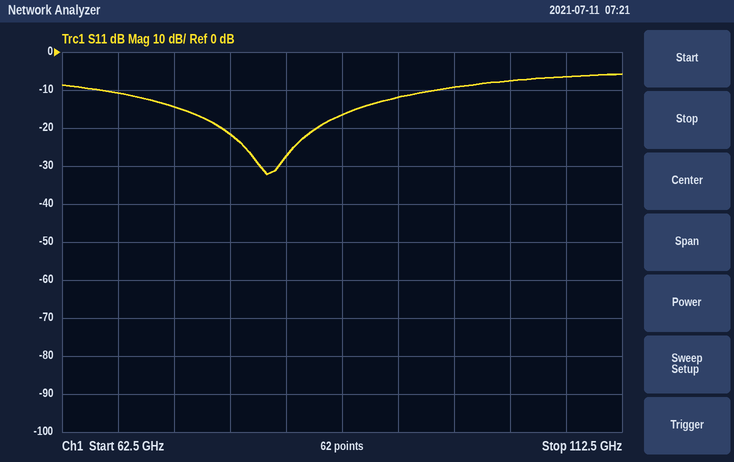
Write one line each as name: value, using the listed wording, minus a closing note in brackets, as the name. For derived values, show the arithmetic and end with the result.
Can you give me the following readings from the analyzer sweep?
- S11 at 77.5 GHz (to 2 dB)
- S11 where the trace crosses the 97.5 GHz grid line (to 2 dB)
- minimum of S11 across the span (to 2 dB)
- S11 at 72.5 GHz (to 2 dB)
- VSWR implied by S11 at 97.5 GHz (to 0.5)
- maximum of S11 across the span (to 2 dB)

S11 at 77.5 GHz: -22 dB
S11 where the trace crosses the 97.5 GHz grid line: -10 dB
minimum of S11 across the span: -32 dB
S11 at 72.5 GHz: -14 dB
VSWR implied by S11 at 97.5 GHz: |Γ| = 10^(-10/20) = 0.3162; VSWR = (1 + 0.3162)/(1 − 0.3162) ≈ 1.92, so 2.0 to the nearest 0.5
maximum of S11 across the span: -6 dB
